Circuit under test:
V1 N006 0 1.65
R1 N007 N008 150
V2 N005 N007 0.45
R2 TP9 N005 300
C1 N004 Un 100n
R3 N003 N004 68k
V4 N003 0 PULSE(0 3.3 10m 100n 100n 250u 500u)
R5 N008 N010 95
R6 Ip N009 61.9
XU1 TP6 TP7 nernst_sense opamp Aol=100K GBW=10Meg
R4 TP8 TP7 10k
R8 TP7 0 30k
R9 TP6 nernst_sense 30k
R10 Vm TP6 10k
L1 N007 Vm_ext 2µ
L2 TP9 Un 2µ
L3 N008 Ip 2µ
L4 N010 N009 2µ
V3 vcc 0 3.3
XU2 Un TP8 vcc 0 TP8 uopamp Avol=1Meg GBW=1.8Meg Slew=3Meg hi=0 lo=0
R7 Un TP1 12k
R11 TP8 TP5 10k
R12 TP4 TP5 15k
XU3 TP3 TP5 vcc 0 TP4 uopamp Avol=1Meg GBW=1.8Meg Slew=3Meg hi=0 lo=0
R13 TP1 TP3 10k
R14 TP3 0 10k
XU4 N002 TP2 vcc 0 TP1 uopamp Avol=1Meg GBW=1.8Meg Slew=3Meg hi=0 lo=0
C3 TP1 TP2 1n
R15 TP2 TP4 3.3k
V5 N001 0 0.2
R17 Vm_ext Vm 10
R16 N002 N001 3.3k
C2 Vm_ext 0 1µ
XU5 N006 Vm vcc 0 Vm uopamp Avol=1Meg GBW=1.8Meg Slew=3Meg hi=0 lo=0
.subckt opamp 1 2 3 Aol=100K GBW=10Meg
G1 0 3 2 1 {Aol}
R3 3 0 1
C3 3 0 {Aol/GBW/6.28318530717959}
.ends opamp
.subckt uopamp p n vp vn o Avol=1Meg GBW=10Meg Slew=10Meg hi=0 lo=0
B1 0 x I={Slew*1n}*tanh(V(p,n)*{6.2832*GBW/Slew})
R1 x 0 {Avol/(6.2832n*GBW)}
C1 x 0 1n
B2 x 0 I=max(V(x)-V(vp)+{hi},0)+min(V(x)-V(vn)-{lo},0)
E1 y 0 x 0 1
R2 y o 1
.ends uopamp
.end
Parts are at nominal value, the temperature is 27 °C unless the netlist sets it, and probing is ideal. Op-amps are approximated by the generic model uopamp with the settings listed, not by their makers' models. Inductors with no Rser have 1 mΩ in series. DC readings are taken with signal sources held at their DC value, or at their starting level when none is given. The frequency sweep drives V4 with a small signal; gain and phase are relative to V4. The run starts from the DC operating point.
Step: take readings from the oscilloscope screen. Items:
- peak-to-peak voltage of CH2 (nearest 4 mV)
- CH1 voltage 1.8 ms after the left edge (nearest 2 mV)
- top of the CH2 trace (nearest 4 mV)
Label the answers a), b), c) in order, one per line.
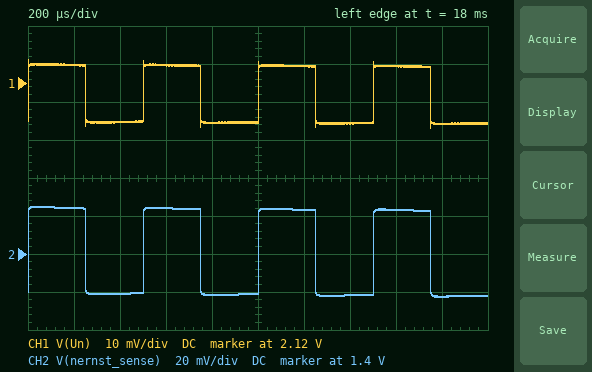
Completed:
a) 48 mV
b) 2.110 V
c) 1.424 V
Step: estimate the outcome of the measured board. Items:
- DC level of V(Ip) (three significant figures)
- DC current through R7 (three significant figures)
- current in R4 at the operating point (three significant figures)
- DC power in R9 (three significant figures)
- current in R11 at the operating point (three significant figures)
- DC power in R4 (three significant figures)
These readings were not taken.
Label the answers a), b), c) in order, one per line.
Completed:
a) 1.65 V
b) 48.6 µA
c) 52.9 µA
d) 1.22 µW
e) 76.6 µA
f) 28.0 µW
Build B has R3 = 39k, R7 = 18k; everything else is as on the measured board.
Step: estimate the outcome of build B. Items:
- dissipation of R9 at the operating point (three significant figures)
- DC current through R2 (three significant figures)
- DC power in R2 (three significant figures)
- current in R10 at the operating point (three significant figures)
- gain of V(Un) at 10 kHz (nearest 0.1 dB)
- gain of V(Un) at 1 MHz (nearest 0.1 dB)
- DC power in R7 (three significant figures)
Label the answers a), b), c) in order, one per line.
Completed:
a) 1.37 µW
b) 32.3 µA
c) 314 nW
d) 6.75 µA
e) -42.1 dB
f) -42.5 dB
g) 18.8 µW
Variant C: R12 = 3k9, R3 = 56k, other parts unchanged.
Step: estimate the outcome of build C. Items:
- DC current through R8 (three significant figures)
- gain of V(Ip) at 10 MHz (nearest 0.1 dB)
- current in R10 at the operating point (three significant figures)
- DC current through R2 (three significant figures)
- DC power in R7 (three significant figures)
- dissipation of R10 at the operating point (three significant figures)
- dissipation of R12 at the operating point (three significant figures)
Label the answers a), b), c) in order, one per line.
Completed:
a) 52.1 µA
b) -53.2 dB
c) 8.72 µA
d) 52.2 µA
e) 32.7 µW
f) 760 nW
g) 71.6 µW
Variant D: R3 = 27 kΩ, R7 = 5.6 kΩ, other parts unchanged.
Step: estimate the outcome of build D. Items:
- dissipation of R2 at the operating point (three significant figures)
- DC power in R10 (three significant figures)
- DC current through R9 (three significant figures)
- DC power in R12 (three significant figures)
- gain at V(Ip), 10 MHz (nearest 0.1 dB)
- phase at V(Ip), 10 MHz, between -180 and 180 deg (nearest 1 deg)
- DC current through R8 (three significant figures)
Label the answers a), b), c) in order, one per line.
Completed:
a) 3.29 µW
b) 257 nW
c) 5.07 µA
d) 89.6 µW
e) -47.2 dB
f) 87 deg
g) 53.3 µA
